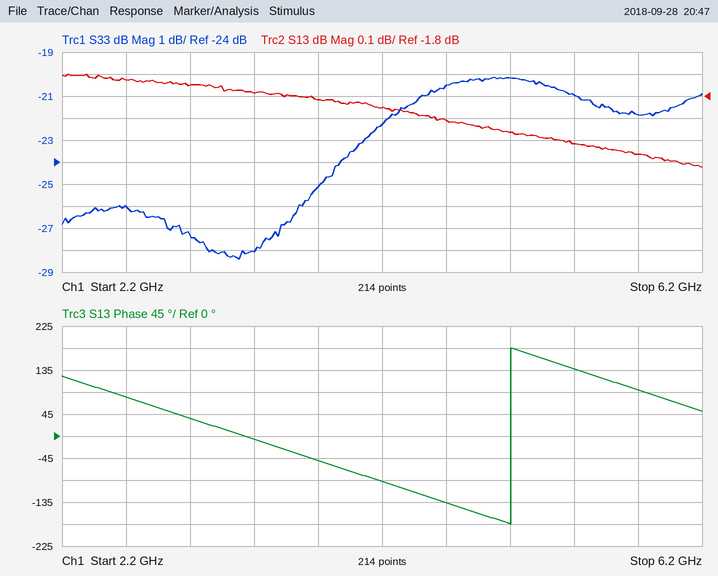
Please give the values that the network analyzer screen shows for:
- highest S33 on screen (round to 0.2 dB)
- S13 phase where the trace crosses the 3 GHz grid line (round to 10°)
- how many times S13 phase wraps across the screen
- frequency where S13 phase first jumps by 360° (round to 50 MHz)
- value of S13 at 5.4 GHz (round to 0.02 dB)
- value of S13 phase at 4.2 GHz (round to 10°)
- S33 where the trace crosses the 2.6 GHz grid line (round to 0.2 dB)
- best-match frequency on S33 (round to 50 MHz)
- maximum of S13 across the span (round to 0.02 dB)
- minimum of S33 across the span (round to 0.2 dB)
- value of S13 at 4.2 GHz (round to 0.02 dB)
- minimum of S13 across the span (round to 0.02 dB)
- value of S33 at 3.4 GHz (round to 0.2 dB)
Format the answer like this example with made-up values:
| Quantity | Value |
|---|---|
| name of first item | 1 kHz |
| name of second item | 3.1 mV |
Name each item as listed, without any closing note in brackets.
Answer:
| Quantity | Value |
|---|---|
| highest S33 on screen | -20.2 dB |
| S13 phase where the trace crosses the 3 GHz grid line | 40° |
| how many times S13 phase wraps across the screen | 1 |
| frequency where S13 phase first jumps by 360° | 5.00 GHz |
| value of S13 at 5.4 GHz | -2.02 dB |
| value of S13 phase at 4.2 GHz | -90° |
| S33 where the trace crosses the 2.6 GHz grid line | -26.0 dB |
| best-match frequency on S33 | 3.30 GHz |
| maximum of S13 across the span | -1.70 dB |
| minimum of S33 across the span | -28.4 dB |
| value of S13 at 4.2 GHz | -1.86 dB |
| minimum of S13 across the span | -2.12 dB |
| value of S33 at 3.4 GHz | -28.0 dB |
